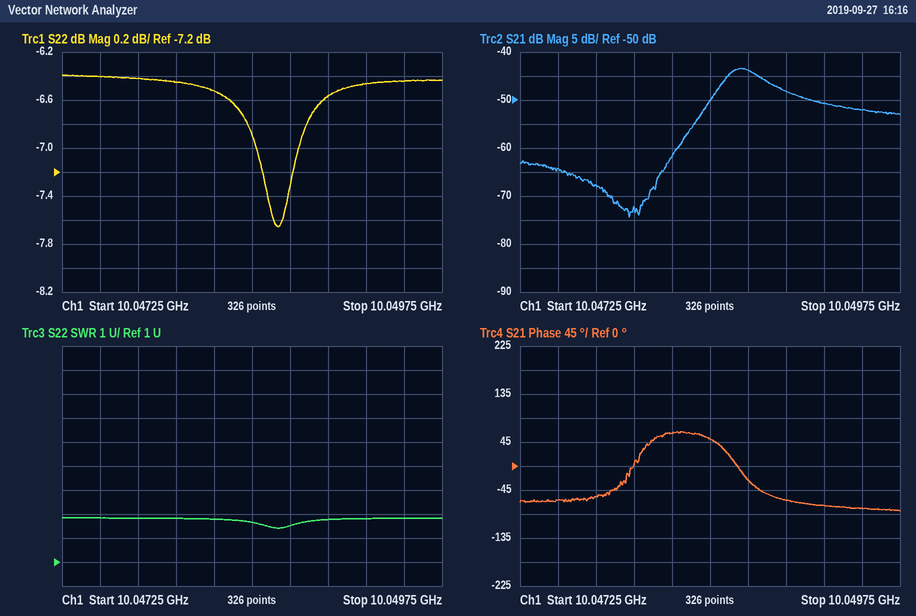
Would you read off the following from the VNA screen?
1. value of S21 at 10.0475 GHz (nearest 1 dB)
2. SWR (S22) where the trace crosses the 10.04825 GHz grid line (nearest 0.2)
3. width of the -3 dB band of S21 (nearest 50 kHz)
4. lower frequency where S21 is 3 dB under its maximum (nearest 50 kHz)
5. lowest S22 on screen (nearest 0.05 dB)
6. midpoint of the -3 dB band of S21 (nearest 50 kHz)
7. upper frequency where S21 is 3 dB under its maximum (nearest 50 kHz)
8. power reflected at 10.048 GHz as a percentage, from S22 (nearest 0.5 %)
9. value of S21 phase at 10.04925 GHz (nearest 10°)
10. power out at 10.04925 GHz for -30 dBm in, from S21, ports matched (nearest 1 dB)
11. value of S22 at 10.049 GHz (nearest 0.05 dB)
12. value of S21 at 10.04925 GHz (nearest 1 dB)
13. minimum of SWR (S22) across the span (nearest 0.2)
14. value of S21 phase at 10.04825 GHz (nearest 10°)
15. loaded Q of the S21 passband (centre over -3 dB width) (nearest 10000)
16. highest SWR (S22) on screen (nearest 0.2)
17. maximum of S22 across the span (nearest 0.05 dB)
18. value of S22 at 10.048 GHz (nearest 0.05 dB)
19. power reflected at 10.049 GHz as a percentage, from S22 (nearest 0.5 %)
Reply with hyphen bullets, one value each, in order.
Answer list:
- -64 dB
- 2.8
- 300 kHz
- 10.04860 GHz
- -7.65 dB
- 10.04875 GHz
- 10.04890 GHz
- 22.5 %
- -70°
- -81 dBm
- -6.55 dB
- -51 dB
- 2.4
- 60°
- 30000
- 2.8
- -6.40 dB
- -6.45 dB
- 22.0 %
